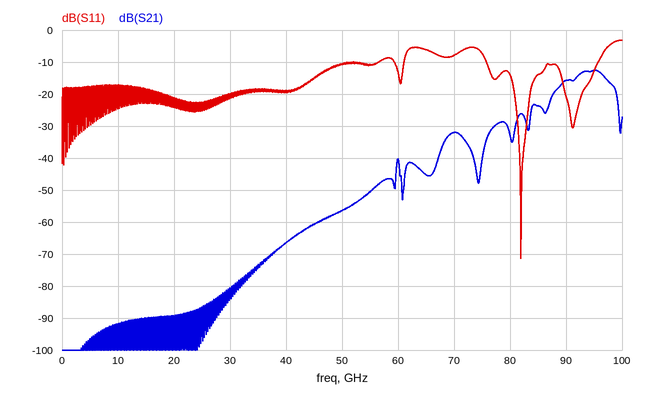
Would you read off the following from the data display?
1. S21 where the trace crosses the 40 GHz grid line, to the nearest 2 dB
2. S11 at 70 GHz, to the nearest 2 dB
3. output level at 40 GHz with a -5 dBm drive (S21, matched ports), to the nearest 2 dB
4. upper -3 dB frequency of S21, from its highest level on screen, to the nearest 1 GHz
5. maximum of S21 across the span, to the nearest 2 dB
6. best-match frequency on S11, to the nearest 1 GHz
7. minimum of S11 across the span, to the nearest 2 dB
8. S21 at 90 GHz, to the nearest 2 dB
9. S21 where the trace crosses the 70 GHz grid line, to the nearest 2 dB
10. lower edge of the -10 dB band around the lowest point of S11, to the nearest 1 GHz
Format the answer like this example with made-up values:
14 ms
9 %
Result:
-66 dB
-8 dB
-72 dBm
97 GHz
-12 dB
82 GHz
-72 dB
-16 dB
-32 dB
76 GHz
